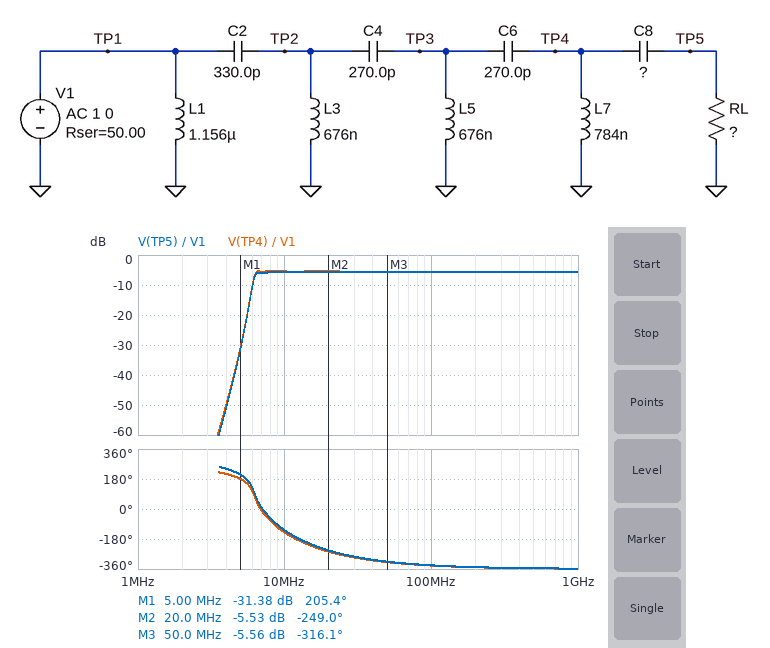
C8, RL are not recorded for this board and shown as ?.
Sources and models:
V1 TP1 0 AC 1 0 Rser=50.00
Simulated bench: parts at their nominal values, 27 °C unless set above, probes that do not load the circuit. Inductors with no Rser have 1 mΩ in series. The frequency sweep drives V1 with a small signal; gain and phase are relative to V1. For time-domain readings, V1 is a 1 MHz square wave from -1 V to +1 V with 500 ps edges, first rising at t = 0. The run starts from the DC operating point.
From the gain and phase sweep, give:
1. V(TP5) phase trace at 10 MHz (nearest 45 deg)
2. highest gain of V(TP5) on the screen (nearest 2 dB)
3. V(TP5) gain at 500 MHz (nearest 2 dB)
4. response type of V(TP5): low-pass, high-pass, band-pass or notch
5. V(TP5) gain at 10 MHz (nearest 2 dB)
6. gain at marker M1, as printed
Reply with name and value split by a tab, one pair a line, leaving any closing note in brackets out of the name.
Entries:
V(TP5) phase trace at 10 MHz	-135 deg
highest gain of V(TP5) on the screen	-6 dB
V(TP5) gain at 500 MHz	-6 dB
response type of V(TP5): low-pass, high-pass, band-pass or notch	high-pass
V(TP5) gain at 10 MHz	-6 dB
gain at marker M1, as printed	-31.38 dB
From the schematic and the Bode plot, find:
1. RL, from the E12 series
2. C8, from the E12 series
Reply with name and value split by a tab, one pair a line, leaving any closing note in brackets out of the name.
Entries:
RL, from the E12 series	56 Ω
C8, from the E12 series	1.2 nF
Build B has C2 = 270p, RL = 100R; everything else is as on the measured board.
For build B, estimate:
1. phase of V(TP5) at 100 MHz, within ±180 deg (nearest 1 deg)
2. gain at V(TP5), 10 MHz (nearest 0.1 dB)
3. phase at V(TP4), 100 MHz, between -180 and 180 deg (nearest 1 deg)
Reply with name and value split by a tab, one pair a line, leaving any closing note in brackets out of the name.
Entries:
phase of V(TP5) at 100 MHz, within ±180 deg	23 deg
gain at V(TP5), 10 MHz	-3.5 dB
phase at V(TP4), 100 MHz, between -180 and 180 deg	22 deg
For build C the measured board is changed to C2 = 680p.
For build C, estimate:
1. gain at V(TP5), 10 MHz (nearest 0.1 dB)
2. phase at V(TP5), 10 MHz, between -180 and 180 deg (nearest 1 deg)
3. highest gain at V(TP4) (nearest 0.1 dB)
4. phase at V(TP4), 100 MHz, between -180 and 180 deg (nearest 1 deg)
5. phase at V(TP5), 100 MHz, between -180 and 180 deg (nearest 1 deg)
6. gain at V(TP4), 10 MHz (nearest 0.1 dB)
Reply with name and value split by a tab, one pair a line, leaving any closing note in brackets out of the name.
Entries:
gain at V(TP5), 10 MHz	-6.7 dB
phase at V(TP5), 10 MHz, between -180 and 180 deg	-146 deg
highest gain at V(TP4)	-5.5 dB
phase at V(TP4), 100 MHz, between -180 and 180 deg	19 deg
phase at V(TP5), 100 MHz, between -180 and 180 deg	21 deg
gain at V(TP4), 10 MHz	-6.5 dB
